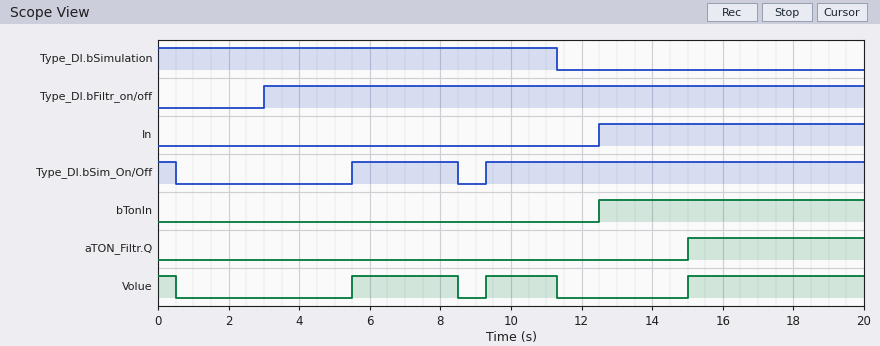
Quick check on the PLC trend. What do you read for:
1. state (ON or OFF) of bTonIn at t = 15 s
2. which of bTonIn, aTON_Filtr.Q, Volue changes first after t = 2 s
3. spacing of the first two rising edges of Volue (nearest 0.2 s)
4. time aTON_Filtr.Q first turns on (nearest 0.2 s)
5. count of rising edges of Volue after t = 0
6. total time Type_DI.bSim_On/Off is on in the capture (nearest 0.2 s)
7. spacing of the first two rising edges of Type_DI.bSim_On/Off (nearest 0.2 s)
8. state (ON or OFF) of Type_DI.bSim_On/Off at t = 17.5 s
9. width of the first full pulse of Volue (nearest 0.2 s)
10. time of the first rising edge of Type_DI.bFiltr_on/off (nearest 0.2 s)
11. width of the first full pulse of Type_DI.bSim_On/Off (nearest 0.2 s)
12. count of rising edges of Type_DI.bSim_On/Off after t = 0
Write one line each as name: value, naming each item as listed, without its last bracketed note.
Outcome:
state (ON or OFF) of bTonIn at t = 15 s: ON
which of bTonIn, aTON_Filtr.Q, Volue changes first after t = 2 s: Volue
spacing of the first two rising edges of Volue: 3.8 s
time aTON_Filtr.Q first turns on: 15.0 s
count of rising edges of Volue after t = 0: 3
total time Type_DI.bSim_On/Off is on in the capture: 14.2 s
spacing of the first two rising edges of Type_DI.bSim_On/Off: 3.8 s
state (ON or OFF) of Type_DI.bSim_On/Off at t = 17.5 s: ON
width of the first full pulse of Volue: 3.0 s
time of the first rising edge of Type_DI.bFiltr_on/off: 3.0 s
width of the first full pulse of Type_DI.bSim_On/Off: 3.0 s
count of rising edges of Type_DI.bSim_On/Off after t = 0: 2
